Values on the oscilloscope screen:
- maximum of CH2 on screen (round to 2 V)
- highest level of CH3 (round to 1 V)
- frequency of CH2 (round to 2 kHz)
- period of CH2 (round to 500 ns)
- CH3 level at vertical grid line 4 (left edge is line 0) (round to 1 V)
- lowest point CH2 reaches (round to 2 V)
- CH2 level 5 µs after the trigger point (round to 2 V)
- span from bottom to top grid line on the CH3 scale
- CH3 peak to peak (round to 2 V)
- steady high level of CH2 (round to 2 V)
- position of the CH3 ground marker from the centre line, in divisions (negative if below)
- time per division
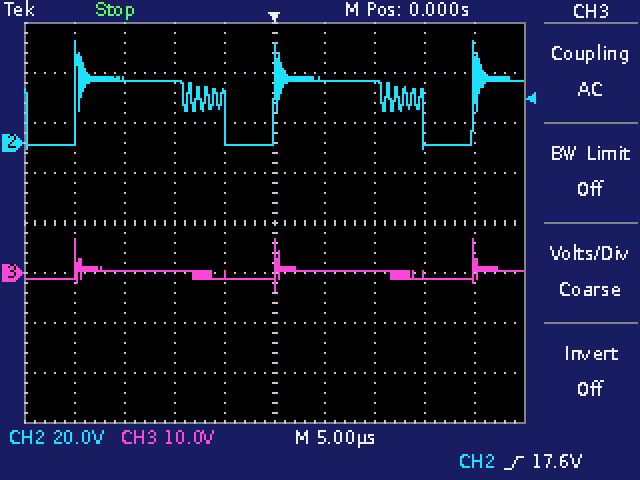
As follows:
40 V
7 V
50 kHz
20.0 µs
0 V
-2 V
24 V
80 V
10 V
24 V
-1.0 div
5 µs
